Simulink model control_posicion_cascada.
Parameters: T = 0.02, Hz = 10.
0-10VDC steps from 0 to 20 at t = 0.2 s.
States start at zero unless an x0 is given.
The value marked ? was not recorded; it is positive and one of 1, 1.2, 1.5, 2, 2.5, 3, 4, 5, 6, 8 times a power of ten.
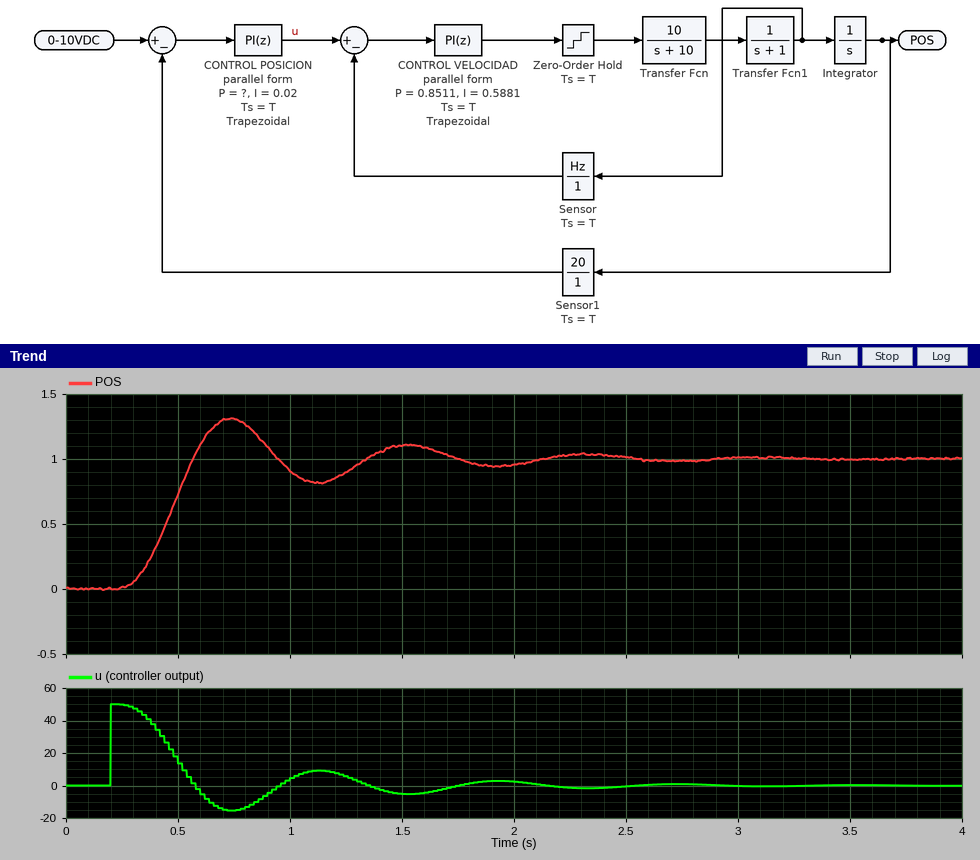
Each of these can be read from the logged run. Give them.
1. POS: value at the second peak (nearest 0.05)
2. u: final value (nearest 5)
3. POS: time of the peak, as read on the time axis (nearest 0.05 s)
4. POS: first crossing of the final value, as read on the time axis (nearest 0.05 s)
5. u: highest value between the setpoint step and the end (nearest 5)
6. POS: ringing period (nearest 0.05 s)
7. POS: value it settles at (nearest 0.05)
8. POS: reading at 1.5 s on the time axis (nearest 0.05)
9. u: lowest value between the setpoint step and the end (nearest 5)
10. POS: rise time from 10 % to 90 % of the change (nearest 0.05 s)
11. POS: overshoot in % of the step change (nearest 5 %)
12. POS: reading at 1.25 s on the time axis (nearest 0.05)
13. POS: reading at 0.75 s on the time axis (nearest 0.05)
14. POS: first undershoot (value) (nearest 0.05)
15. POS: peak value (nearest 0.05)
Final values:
1.10
0
0.75 s
0.55 s
50
0.80 s
1.00
1.10
-15
0.20 s
30 %
0.90
1.30
0.80
1.30
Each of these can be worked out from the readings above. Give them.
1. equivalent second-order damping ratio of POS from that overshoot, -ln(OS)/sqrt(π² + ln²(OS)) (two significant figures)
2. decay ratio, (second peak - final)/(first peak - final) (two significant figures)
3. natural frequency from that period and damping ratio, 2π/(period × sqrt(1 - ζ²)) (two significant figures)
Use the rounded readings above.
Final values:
0.36
0.33
8.4 rad/s
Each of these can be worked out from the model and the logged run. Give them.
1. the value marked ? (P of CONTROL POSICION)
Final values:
2.5
